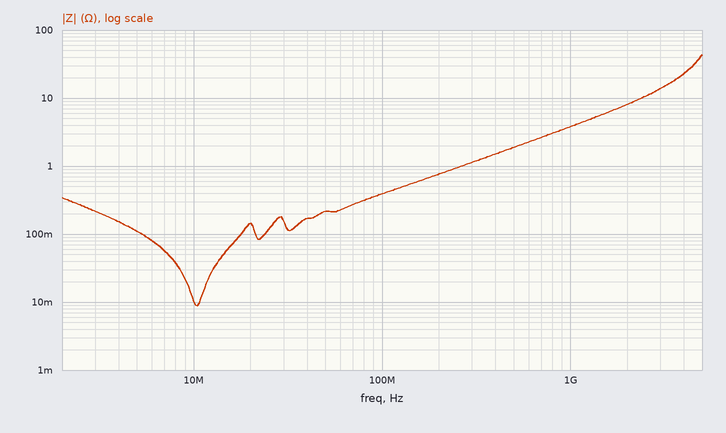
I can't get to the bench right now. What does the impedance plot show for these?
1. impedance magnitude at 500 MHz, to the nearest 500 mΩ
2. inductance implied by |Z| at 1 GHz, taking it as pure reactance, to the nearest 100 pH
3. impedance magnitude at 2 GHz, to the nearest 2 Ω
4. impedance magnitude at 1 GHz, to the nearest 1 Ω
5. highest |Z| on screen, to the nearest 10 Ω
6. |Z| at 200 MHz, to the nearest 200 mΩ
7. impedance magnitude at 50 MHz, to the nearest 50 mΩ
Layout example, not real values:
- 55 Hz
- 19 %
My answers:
- 2.0 Ω
- 600 pH
- 8 Ω
- 4 Ω
- 40 Ω
- 800 mΩ
- 200 mΩ
